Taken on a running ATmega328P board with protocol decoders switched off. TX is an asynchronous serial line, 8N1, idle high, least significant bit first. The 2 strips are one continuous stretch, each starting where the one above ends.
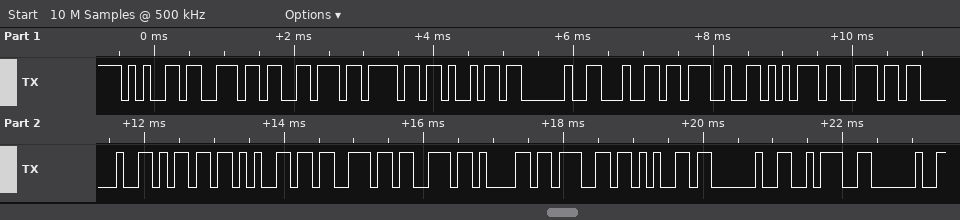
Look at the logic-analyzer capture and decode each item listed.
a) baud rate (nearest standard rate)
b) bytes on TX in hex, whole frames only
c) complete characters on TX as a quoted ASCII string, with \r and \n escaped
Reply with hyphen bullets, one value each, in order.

- 9600 baud
- 65 6E 76 6F 69 20 64 27 75 6E 20 6D 65 73 73 61 67 65 20 3A 20
- "envoi d'un message : "
